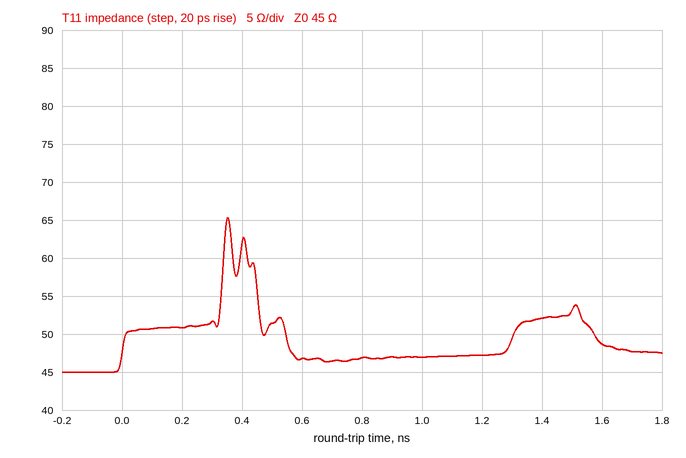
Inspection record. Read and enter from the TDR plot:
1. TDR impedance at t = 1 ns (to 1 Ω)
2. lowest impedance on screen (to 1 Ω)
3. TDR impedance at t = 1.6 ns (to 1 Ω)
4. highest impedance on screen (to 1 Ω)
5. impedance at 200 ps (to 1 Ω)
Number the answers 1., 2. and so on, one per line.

1. 47 Ω
2. 45 Ω
3. 49 Ω
4. 65 Ω
5. 51 Ω
